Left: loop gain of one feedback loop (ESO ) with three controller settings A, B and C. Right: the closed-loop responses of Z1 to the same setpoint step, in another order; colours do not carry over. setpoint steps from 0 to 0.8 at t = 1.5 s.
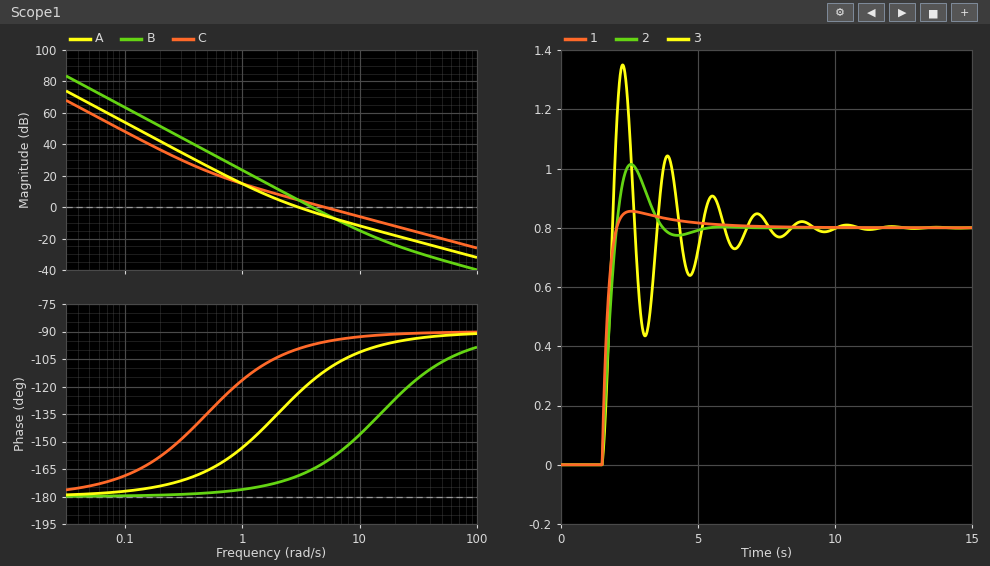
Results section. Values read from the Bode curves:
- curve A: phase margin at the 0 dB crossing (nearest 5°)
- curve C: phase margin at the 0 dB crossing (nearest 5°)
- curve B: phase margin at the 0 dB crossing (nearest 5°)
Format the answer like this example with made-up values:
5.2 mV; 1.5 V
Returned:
55°; 85°; 15°
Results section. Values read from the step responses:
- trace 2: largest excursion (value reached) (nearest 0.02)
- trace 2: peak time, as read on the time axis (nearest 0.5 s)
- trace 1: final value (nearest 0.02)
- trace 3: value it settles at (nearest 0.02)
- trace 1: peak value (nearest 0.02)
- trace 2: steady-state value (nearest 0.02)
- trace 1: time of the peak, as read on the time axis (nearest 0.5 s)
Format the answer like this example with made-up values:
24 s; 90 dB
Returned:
1.02; 2.5 s; 0.80; 0.80; 0.86; 0.80; 2.5 s
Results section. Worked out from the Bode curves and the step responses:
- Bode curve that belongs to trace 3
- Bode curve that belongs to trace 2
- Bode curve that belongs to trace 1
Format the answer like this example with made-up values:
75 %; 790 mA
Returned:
B; A; C
